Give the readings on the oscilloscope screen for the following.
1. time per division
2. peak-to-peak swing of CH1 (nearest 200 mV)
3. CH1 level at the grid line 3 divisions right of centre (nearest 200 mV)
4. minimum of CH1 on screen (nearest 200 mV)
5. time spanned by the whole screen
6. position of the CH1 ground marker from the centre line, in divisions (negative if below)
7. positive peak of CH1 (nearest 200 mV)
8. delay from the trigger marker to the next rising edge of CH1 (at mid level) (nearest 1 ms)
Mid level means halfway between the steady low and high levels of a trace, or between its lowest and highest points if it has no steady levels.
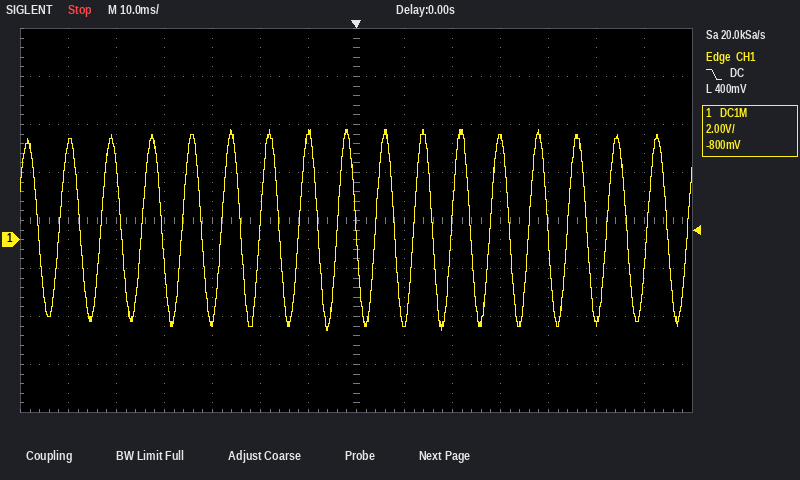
10 ms
8.4 V
4.2 V
-3.8 V
140 ms
-0.4 div
4.6 V
4 ms
